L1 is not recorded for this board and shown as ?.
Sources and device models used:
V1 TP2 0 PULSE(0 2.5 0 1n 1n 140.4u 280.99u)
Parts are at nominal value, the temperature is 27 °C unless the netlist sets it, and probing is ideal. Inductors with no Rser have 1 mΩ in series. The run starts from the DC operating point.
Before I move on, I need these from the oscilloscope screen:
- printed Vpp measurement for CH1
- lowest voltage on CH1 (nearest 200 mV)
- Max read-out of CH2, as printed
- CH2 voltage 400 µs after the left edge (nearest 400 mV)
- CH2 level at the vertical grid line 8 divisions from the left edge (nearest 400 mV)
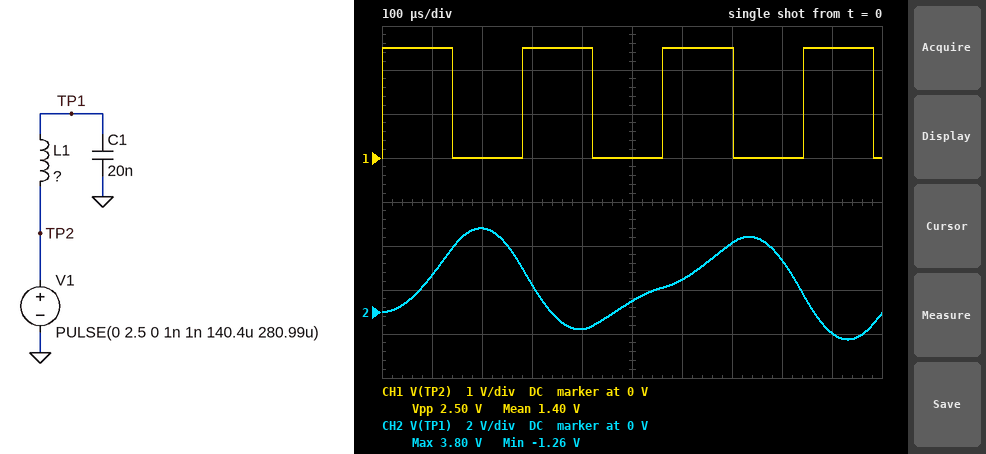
2.50 V
0 V
3.80 V
-800 mV
2.4 V
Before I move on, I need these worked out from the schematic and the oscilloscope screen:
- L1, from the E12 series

330 mH
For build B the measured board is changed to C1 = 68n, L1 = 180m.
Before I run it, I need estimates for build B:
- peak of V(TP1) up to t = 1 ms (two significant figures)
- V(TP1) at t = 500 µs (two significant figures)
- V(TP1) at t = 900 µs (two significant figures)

3.0 V
880 mV
2.2 V
